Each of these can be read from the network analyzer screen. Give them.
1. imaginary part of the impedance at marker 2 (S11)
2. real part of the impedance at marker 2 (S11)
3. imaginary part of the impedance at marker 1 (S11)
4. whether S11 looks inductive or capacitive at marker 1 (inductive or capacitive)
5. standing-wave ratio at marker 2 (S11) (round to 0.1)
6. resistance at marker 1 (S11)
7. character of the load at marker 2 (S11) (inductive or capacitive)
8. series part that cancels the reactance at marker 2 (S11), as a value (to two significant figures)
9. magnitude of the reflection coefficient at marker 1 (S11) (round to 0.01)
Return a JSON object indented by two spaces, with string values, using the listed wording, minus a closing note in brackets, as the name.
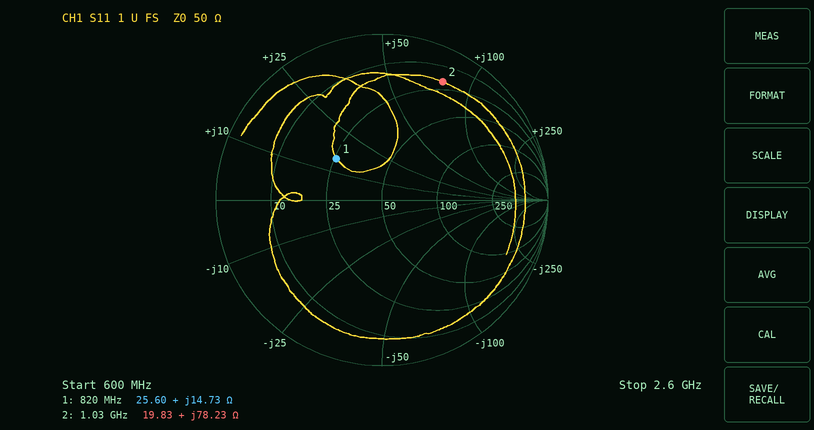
{
  "imaginary part of the impedance at marker 2": "+78.23 Ω",
  "real part of the impedance at marker 2": "19.83 Ω",
  "imaginary part of the impedance at marker 1": "+14.73 Ω",
  "whether S11 looks inductive or capacitive at marker 1": "inductive",
  "standing-wave ratio at marker 2 (S11)": "9.0",
  "resistance at marker 1": "25.60 Ω",
  "character of the load at marker 2 (S11)": "inductive",
  "series part that cancels the reactance at marker 2 (S11), as a value": "2.0 pF",
  "magnitude of the reflection coefficient at marker 1 (S11)": "0.37"
}
